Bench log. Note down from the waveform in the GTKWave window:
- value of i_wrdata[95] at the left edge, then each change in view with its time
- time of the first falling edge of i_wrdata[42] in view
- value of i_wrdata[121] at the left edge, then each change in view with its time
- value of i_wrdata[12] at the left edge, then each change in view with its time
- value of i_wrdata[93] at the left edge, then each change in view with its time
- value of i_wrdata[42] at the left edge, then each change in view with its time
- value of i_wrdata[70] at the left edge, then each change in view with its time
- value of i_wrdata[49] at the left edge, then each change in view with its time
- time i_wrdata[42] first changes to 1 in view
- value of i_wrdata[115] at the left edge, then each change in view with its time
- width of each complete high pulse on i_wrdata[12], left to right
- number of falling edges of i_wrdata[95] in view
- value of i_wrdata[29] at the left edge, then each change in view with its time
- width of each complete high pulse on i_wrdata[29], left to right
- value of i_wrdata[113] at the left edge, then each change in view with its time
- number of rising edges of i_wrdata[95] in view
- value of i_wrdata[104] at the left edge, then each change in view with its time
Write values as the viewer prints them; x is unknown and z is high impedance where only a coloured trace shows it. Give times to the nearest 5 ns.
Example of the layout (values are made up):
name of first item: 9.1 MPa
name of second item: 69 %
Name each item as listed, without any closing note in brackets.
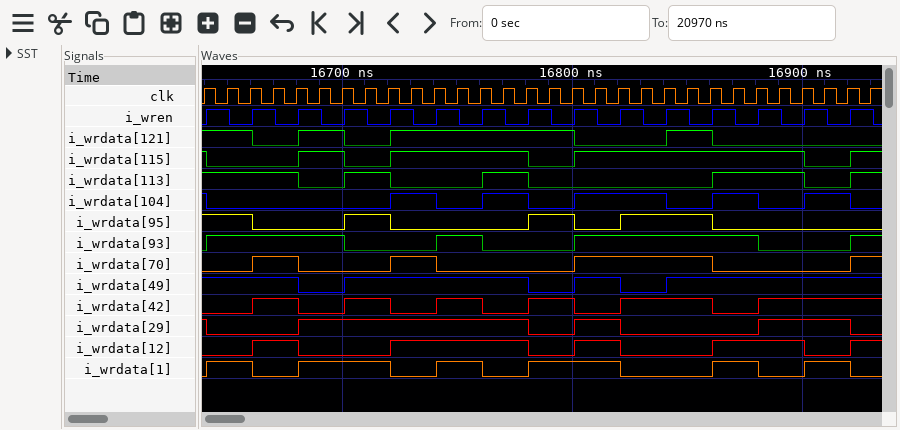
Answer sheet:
value of i_wrdata[95] at the left edge, then each change in view with its time: 1, 0 at 16660 ns, 1 at 16700 ns, 0 at 16720 ns, 1 at 16780 ns, 0 at 16800 ns, 1 at 16820 ns, 0 at 16860 ns
time of the first falling edge of i_wrdata[42] in view: 16680 ns
value of i_wrdata[121] at the left edge, then each change in view with its time: 1, 0 at 16660 ns, 1 at 16680 ns, 0 at 16700 ns, 1 at 16720 ns, 0 at 16800 ns, 1 at 16840 ns, 0 at 16860 ns
value of i_wrdata[12] at the left edge, then each change in view with its time: 0, 1 at 16660 ns, 0 at 16680 ns, 1 at 16720 ns, 0 at 16780 ns, 1 at 16800 ns, 0 at 16820 ns, 1 at 16860 ns, 0 at 16900 ns, 1 at 16920 ns
value of i_wrdata[93] at the left edge, then each change in view with its time: 0, 1 at 16640 ns, 0 at 16700 ns, 1 at 16740 ns, 0 at 16760 ns, 1 at 16800 ns, 0 at 16880 ns, 1 at 16920 ns
value of i_wrdata[42] at the left edge, then each change in view with its time: 0, 1 at 16660 ns, 0 at 16680 ns, 1 at 16700 ns, 0 at 16720 ns, 1 at 16740 ns, 0 at 16760 ns, 1 at 16780 ns, 0 at 16800 ns, 1 at 16820 ns, 0 at 16860 ns, 1 at 16880 ns
value of i_wrdata[70] at the left edge, then each change in view with its time: 0, 1 at 16660 ns, 0 at 16680 ns, 1 at 16720 ns, 0 at 16740 ns, 1 at 16800 ns, 0 at 16860 ns, 1 at 16920 ns
value of i_wrdata[49] at the left edge, then each change in view with its time: 1, 0 at 16680 ns, 1 at 16700 ns, 0 at 16780 ns, 1 at 16800 ns, 0 at 16820 ns, 1 at 16840 ns
time i_wrdata[42] first changes to 1 in view: 16660 ns
value of i_wrdata[115] at the left edge, then each change in view with its time: 1, 0 at 16640 ns, 1 at 16680 ns, 0 at 16700 ns, 1 at 16720 ns, 0 at 16780 ns, 1 at 16800 ns, 0 at 16900 ns, 1 at 16920 ns
width of each complete high pulse on i_wrdata[12], left to right: 20 ns, 60 ns, 20 ns, 40 ns
number of falling edges of i_wrdata[95] in view: 4
value of i_wrdata[29] at the left edge, then each change in view with its time: 1, 0 at 16640 ns, 1 at 16680 ns, 0 at 16780 ns, 1 at 16800 ns, 0 at 16820 ns, 1 at 16880 ns, 0 at 16920 ns
width of each complete high pulse on i_wrdata[29], left to right: 100 ns, 20 ns, 40 ns
value of i_wrdata[113] at the left edge, then each change in view with its time: 1, 0 at 16680 ns, 1 at 16700 ns, 0 at 16720 ns, 1 at 16760 ns, 0 at 16780 ns, 1 at 16860 ns, 0 at 16900 ns, 1 at 16920 ns
number of rising edges of i_wrdata[95] in view: 3
value of i_wrdata[104] at the left edge, then each change in view with its time: 1, 0 at 16640 ns, 1 at 16720 ns, 0 at 16740 ns, 1 at 16760 ns, 0 at 16780 ns, 1 at 16800 ns, 0 at 16840 ns, 1 at 16860 ns, 0 at 16880 ns, 1 at 16900 ns, 0 at 16920 ns
